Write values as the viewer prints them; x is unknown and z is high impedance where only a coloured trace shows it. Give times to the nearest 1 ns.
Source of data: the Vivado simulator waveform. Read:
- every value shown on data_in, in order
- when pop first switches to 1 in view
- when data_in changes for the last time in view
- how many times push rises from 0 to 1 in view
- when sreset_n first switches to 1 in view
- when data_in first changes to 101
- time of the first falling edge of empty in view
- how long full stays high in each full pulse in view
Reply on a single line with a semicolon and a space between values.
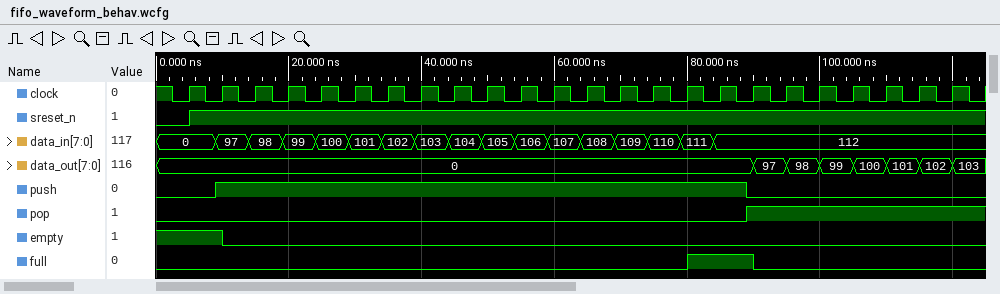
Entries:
0, 97, 98, 99, 100, 101, 102, 103, 104, 105, 106, 107, 108, 109, 110, 111, 112; 89 ns; 84 ns; 1; 5 ns; 29 ns; 10 ns; 10 ns
